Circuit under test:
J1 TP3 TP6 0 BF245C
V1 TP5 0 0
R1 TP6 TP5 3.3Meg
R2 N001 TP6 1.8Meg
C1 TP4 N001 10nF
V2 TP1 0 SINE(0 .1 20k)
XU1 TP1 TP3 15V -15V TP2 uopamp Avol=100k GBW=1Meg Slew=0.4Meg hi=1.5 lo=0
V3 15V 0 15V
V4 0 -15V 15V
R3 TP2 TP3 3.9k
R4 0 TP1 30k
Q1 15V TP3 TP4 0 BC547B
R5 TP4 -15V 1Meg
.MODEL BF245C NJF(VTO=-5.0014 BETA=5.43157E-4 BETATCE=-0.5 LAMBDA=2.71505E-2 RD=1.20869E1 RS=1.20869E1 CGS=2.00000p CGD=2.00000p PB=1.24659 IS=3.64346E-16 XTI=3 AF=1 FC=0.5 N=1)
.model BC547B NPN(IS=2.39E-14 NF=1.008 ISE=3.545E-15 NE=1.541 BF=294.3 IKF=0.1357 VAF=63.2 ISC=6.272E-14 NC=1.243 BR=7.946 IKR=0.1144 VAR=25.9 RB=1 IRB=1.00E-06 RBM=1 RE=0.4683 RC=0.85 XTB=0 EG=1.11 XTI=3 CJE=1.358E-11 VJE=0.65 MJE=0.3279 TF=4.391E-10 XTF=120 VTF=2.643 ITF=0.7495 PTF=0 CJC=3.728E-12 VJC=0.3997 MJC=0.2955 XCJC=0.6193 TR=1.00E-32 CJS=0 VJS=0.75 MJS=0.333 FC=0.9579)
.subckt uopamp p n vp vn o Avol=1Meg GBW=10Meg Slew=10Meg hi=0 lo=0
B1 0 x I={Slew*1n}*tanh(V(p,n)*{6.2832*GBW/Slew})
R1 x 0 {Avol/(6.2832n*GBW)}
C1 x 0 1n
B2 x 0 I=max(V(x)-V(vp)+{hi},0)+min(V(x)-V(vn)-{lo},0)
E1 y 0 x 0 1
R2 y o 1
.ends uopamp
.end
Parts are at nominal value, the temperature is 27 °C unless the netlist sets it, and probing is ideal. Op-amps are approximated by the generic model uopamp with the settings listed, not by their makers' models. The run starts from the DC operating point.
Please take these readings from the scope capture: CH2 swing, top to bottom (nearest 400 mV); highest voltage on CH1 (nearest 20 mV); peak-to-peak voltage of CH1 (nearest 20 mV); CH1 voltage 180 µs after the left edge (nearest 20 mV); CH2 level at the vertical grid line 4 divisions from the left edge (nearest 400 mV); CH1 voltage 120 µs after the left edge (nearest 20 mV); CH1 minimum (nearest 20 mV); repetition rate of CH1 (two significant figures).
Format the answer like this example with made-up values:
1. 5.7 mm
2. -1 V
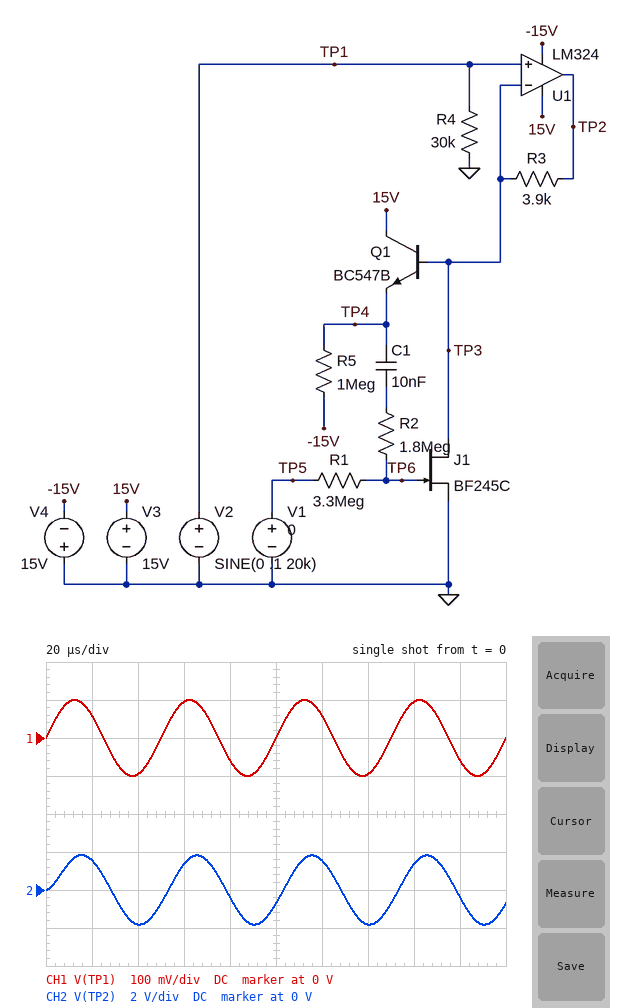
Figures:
1. 3.6 V
2. 100 mV
3. 200 mV
4. -60 mV
5. -400 mV
6. 60 mV
7. -100 mV
8. 20 kHz
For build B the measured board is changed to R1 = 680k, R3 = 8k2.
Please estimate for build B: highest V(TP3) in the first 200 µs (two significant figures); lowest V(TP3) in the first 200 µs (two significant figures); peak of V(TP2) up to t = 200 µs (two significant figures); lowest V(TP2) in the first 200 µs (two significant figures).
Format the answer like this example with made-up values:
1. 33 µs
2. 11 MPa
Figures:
1. 78 mV
2. -71 mV
3. 3.2 V
4. -2.9 V
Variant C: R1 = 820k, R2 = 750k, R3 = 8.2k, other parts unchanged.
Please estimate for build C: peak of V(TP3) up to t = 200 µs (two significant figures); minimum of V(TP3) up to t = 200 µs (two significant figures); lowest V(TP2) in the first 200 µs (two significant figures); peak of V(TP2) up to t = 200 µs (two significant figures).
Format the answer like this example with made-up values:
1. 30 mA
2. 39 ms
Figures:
1. 78 mV
2. -71 mV
3. -2.9 V
4. 3.2 V
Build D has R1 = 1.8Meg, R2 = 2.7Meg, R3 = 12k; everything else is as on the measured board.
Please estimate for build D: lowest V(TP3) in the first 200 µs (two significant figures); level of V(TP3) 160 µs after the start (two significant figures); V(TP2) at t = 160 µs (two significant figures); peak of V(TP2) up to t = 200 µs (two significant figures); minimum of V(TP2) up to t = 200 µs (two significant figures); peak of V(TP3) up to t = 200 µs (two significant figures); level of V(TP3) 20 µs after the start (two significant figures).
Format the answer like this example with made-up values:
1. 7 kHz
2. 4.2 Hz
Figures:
1. -54 mV
2. 11 mV
3. 650 mV
4. 3.9 V
5. -3.2 V
6. 67 mV
7. 66 mV
